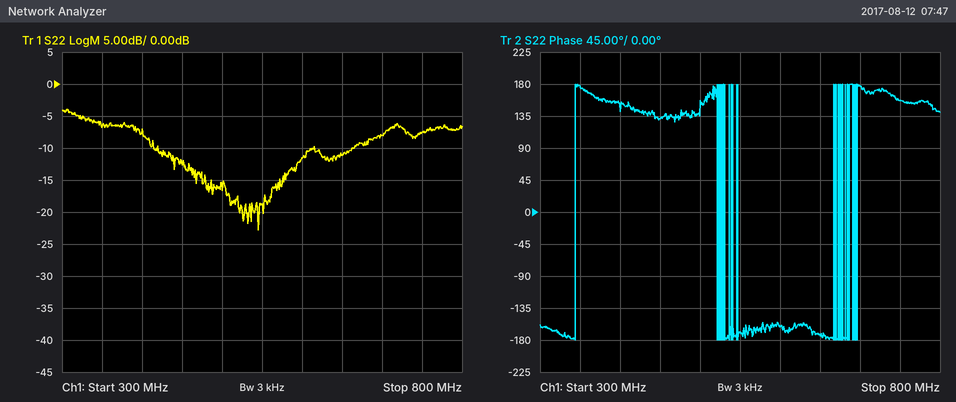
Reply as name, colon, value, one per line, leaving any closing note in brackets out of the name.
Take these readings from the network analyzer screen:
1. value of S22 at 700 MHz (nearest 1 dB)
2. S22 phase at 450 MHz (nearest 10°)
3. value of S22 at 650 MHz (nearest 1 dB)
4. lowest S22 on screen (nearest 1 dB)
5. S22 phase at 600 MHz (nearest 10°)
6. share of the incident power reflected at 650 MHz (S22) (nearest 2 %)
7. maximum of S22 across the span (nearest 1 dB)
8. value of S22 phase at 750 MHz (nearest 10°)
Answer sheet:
value of S22 at 700 MHz: -8 dB
S22 phase at 450 MHz: 130°
value of S22 at 650 MHz: -11 dB
lowest S22 on screen: -23 dB
S22 phase at 600 MHz: -160°
share of the incident power reflected at 650 MHz (S22): 8 %
maximum of S22 across the span: -4 dB
value of S22 phase at 750 MHz: 160°
